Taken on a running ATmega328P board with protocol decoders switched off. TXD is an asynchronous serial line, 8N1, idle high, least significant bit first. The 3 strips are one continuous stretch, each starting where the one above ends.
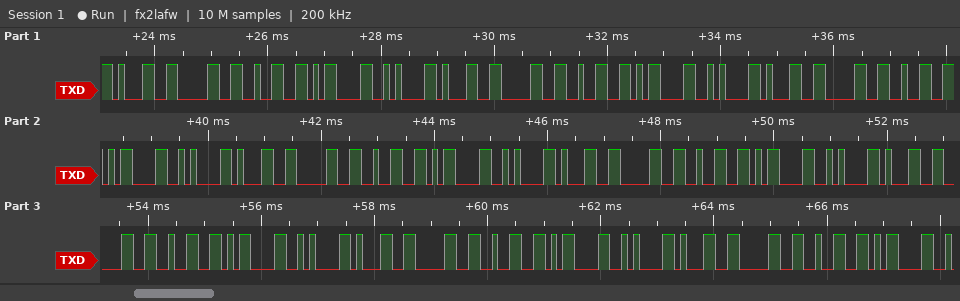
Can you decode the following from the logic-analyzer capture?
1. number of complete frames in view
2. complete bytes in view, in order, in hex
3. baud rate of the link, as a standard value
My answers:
39
31 30 32 0D 0A 31 30 32 0D 0A 31 30 32 0D 0A 31 30 32 0D 0A 31 30 32 0D 0A 31 30 32 0D 0A 31 30 32 0D 0A 31 30 32 0D
9600 baud
